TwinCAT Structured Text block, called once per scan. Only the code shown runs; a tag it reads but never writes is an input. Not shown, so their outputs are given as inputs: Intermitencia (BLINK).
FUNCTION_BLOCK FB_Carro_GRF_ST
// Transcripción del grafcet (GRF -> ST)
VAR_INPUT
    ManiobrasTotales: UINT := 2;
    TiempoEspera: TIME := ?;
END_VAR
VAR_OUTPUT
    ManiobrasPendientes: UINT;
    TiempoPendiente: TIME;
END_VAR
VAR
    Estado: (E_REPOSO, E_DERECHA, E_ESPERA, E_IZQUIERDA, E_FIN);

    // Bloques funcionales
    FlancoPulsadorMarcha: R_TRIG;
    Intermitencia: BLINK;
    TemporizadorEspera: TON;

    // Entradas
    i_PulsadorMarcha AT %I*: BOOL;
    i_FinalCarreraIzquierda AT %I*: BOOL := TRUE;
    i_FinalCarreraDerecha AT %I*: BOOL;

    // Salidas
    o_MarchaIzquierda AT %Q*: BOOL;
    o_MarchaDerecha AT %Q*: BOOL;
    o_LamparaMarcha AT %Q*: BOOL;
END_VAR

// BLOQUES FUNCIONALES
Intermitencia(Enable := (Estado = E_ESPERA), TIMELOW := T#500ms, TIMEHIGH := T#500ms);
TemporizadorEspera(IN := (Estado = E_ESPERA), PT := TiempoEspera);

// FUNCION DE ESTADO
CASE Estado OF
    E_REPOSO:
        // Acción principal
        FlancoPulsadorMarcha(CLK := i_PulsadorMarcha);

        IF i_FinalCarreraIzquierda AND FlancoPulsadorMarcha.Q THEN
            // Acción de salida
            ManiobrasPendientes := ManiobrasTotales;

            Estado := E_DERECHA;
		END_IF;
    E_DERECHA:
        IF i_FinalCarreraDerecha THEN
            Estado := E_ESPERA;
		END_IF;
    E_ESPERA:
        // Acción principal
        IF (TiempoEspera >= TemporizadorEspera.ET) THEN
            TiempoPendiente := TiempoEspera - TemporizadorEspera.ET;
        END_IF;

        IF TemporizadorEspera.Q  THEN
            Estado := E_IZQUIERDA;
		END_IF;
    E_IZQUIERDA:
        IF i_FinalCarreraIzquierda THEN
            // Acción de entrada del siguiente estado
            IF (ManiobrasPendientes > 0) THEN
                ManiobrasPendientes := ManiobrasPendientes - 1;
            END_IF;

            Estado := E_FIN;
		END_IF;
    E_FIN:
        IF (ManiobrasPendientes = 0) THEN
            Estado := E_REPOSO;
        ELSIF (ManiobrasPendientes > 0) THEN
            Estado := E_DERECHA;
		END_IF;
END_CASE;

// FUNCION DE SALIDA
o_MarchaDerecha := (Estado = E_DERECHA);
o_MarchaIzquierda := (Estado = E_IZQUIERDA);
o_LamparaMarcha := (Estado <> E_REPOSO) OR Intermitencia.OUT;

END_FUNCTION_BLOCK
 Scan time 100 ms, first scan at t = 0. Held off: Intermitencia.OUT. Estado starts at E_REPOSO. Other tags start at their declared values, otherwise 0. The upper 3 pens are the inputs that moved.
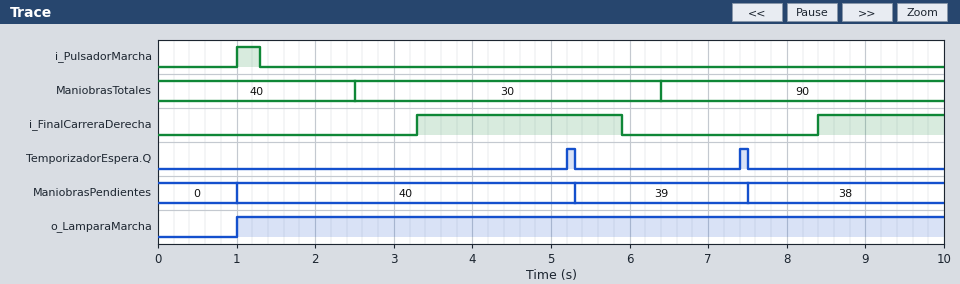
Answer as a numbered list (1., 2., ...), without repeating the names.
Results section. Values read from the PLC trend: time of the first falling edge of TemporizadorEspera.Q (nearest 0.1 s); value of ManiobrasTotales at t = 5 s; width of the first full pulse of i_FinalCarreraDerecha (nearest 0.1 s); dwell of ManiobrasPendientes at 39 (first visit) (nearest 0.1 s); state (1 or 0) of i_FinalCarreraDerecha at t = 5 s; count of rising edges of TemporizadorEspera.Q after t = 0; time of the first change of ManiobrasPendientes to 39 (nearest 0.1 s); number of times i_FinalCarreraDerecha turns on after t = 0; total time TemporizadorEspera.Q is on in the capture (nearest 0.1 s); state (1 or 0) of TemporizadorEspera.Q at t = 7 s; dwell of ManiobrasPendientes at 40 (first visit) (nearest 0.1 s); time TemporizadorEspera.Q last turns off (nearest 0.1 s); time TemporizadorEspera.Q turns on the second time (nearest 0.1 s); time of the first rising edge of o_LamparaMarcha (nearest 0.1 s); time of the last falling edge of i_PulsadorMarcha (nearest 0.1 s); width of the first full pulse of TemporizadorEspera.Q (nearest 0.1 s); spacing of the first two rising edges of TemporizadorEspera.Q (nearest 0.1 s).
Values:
1. 5.3 s
2. 30
3. 2.6 s
4. 2.2 s
5. 1
6. 2
7. 5.3 s
8. 2
9. 0.2 s
10. 0
11. 4.3 s
12. 7.5 s
13. 7.4 s
14. 1.0 s
15. 1.3 s
16. 0.1 s
17. 2.2 s
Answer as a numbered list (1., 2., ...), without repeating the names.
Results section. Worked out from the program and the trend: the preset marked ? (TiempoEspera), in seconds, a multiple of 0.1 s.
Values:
1. 1.8 s
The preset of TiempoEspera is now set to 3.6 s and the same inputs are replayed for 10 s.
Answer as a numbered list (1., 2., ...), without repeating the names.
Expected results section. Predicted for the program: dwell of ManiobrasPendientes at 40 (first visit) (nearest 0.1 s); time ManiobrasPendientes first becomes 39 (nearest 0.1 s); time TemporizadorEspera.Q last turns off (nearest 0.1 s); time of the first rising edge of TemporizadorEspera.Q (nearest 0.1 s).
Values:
1. 6.1 s
2. 7.1 s
3. 7.1 s
4. 7.0 s
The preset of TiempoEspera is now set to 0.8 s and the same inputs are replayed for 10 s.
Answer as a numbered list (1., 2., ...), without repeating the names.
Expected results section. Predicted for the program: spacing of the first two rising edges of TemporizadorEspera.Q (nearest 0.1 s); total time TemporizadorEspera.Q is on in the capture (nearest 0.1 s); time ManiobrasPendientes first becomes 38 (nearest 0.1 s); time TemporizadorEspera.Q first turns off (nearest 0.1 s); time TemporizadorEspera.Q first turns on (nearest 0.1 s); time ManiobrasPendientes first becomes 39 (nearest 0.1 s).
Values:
1. 1.2 s
2. 0.4 s
3. 5.5 s
4. 4.3 s
5. 4.2 s
6. 4.3 s
